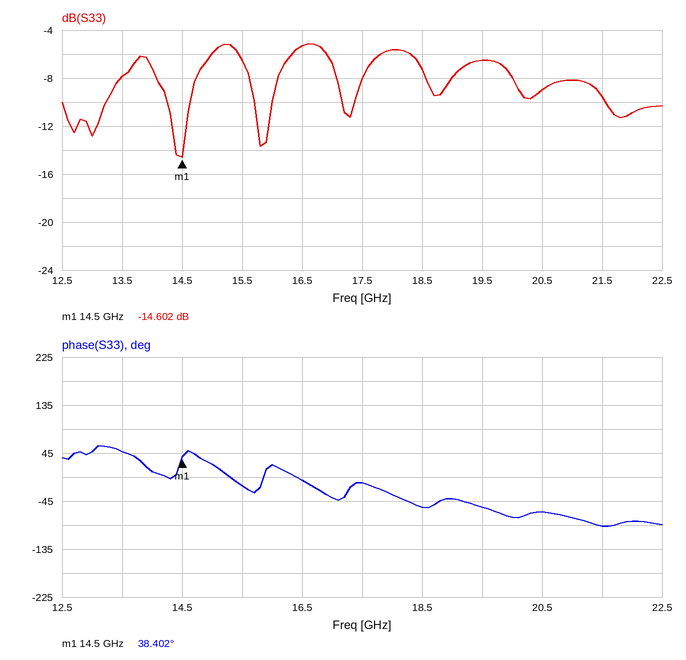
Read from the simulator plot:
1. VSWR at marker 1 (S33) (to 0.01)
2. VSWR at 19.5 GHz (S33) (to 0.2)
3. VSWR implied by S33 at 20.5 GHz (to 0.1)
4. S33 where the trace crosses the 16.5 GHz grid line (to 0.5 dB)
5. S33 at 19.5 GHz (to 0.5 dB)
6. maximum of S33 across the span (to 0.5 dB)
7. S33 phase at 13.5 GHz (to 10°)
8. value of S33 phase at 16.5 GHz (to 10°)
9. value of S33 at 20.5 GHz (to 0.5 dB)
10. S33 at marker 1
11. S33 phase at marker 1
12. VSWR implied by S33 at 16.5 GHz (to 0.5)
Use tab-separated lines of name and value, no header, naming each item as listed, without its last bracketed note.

VSWR at marker 1 (S33)	1.46
VSWR at 19.5 GHz (S33)	2.8
VSWR implied by S33 at 20.5 GHz	2.1
S33 where the trace crosses the 16.5 GHz grid line	-5.5 dB
S33 at 19.5 GHz	-6.5 dB
maximum of S33 across the span	-5.0 dB
S33 phase at 13.5 GHz	50°
value of S33 phase at 16.5 GHz	-10°
value of S33 at 20.5 GHz	-9.0 dB
S33 at marker 1	-14.602 dB
S33 phase at marker 1	38.402°
VSWR implied by S33 at 16.5 GHz	3.5
